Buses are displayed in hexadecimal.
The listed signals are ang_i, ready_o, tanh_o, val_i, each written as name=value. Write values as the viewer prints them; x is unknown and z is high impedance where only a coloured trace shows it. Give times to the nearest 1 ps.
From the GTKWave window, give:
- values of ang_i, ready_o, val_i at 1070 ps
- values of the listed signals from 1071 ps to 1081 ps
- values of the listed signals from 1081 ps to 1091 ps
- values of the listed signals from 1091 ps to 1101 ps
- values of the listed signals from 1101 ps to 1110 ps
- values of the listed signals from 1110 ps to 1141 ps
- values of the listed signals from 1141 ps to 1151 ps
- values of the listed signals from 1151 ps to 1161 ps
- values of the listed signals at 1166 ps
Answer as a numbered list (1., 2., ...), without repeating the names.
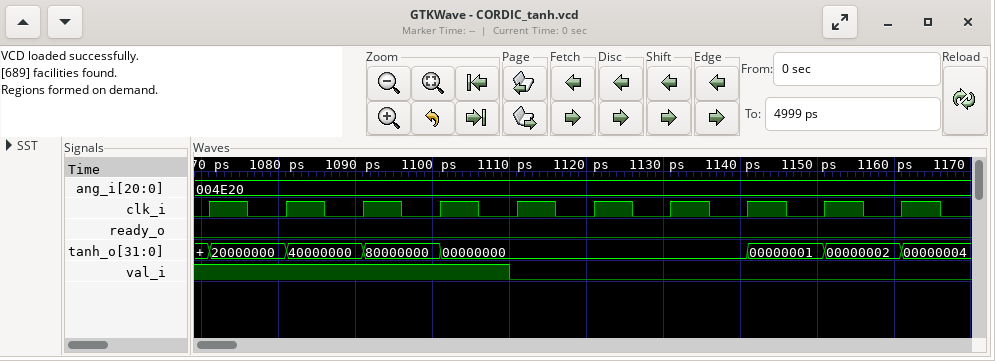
1. ang_i=004E20, ready_o=0, val_i=1
2. ang_i=004E20, ready_o=0, tanh_o=20000000, val_i=1
3. ang_i=004E20, ready_o=0, tanh_o=40000000, val_i=1
4. ang_i=004E20, ready_o=0, tanh_o=80000000, val_i=1
5. ang_i=004E20, ready_o=0, tanh_o=00000000, val_i=1
6. ang_i=004E20, ready_o=0, tanh_o=00000000, val_i=0
7. ang_i=004E20, ready_o=0, tanh_o=00000001, val_i=0
8. ang_i=004E20, ready_o=0, tanh_o=00000002, val_i=0
9. ang_i=004E20, ready_o=0, tanh_o=00000004, val_i=0
